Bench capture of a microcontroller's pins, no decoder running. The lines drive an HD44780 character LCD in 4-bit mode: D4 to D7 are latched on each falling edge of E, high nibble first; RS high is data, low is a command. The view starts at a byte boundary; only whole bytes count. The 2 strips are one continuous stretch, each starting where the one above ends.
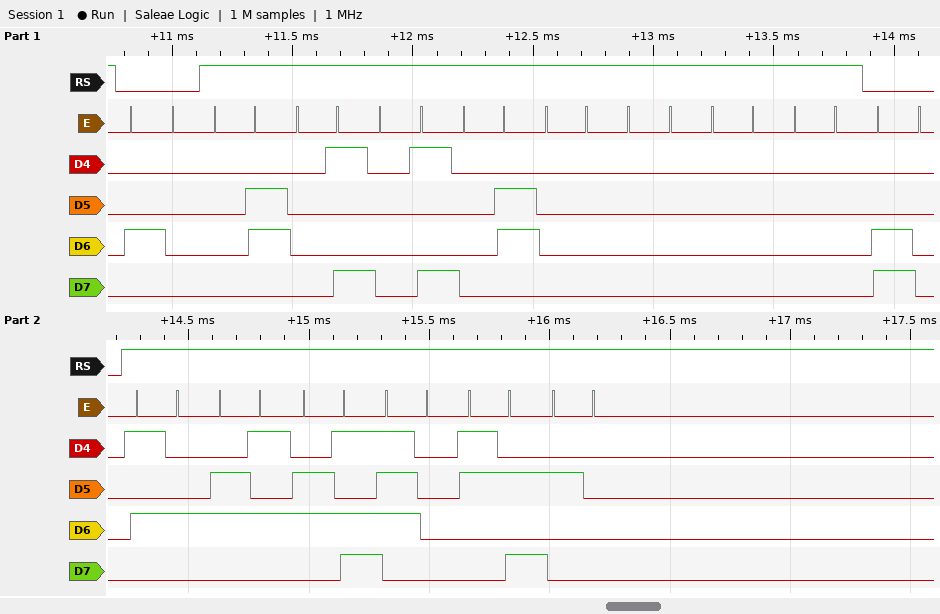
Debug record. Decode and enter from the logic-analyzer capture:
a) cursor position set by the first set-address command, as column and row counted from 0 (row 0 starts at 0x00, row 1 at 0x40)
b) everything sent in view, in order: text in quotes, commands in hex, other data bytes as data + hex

column 0, row 1
0x40 data 06 09 09 06 00 00 00 00 0xC0 "Temp: "
